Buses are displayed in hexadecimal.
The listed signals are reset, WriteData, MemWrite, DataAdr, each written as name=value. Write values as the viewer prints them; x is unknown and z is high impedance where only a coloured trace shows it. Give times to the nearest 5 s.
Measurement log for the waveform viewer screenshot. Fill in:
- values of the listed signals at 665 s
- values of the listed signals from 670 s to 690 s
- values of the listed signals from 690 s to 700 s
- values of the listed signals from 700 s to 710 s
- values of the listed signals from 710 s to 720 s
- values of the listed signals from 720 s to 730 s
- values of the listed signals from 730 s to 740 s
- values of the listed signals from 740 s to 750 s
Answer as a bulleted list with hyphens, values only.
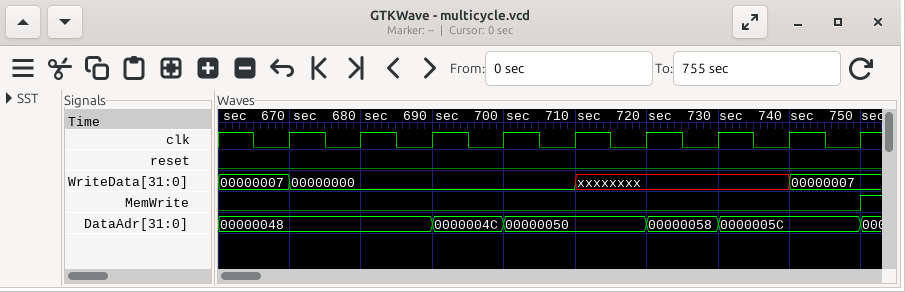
- reset=0, WriteData=00000007, MemWrite=0, DataAdr=00000048
- reset=0, WriteData=00000000, MemWrite=0, DataAdr=00000048
- reset=0, WriteData=00000000, MemWrite=0, DataAdr=0000004C
- reset=0, WriteData=00000000, MemWrite=0, DataAdr=00000050
- reset=0, WriteData=xxxxxxxx, MemWrite=0, DataAdr=00000050
- reset=0, WriteData=xxxxxxxx, MemWrite=0, DataAdr=00000058
- reset=0, WriteData=xxxxxxxx, MemWrite=0, DataAdr=0000005C
- reset=0, WriteData=00000007, MemWrite=0, DataAdr=0000005C
